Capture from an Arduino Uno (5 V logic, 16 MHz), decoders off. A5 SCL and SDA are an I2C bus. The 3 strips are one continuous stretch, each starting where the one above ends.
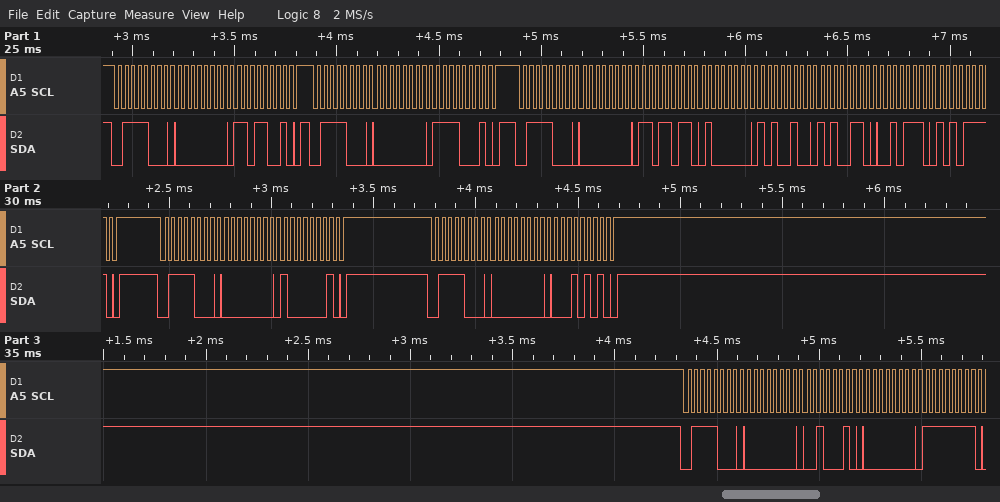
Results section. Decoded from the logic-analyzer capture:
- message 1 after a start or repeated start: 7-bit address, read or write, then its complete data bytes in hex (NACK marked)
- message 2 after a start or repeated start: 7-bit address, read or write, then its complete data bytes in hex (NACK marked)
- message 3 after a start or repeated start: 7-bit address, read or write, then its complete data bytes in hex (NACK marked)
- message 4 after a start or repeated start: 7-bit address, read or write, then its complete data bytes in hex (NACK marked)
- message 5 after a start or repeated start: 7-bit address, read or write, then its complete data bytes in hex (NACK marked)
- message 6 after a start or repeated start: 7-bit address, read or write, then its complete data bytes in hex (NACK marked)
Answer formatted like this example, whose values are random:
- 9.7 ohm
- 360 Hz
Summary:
- 0x3C write: 00 D9
- 0x3C write: 00 F1
- 0x3C write: 00 DB 40 A4 A6 2E AF
- 0x3C write: 00 81
- 0x3C write: 00 15
- 0x3C write: 00 22 00 FF
